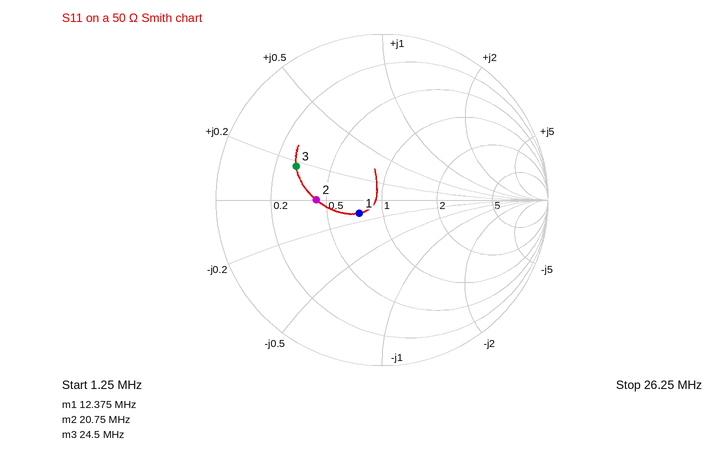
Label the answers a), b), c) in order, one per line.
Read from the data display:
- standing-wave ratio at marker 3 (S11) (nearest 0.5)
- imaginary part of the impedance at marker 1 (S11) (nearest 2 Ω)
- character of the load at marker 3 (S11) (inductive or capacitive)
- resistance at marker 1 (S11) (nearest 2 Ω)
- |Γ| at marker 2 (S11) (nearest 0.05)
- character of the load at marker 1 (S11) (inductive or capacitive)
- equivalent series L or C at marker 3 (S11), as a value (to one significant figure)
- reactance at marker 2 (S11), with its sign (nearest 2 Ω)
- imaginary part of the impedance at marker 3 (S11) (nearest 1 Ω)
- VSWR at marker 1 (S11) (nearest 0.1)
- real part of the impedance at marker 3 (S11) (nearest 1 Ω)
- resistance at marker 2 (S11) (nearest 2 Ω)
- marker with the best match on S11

a) 3.5
b) -6 Ω
c) inductive
d) 38 Ω
e) 0.40
f) capacitive
g) 60 nH
h) 0 Ω
i) +9 Ω
j) 1.4
k) 15 Ω
l) 22 Ω
m) marker 1
